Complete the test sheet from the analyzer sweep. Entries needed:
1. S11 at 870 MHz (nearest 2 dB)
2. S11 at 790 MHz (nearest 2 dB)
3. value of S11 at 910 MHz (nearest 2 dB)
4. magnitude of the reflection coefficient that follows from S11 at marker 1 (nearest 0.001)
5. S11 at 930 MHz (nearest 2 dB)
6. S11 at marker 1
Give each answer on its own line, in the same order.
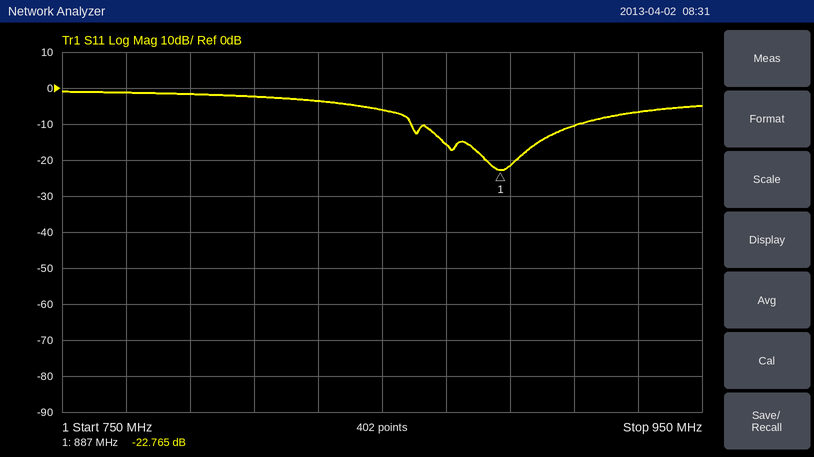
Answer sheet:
-16 dB
-2 dB
-10 dB
0.073
-6 dB
-22.765 dB
